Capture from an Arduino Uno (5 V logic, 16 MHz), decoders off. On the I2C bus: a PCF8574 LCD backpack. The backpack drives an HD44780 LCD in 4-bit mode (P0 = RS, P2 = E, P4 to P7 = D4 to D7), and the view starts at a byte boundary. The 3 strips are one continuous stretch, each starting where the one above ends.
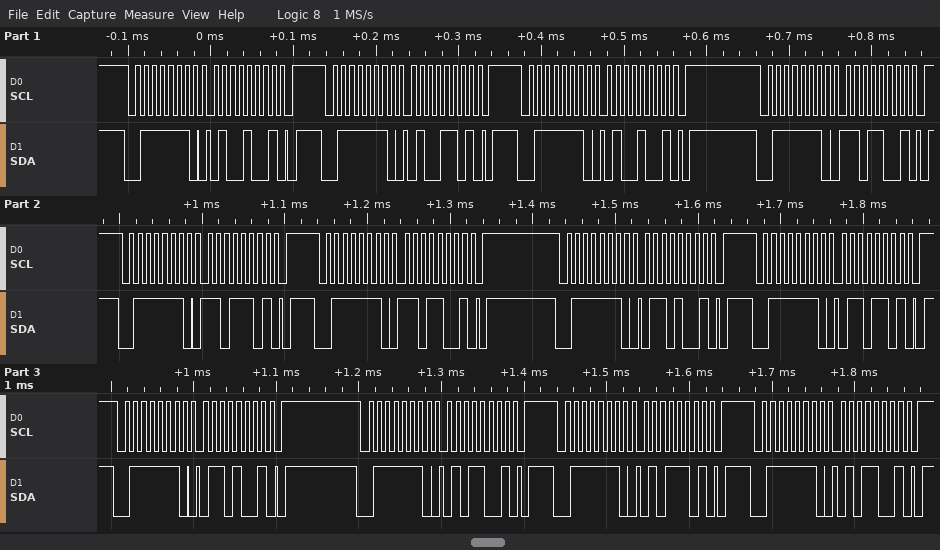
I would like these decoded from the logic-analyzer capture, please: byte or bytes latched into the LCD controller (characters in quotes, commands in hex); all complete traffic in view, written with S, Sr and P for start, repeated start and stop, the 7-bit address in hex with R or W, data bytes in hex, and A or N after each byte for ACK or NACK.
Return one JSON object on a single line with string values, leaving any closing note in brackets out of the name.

{"byte or bytes latched into the LCD controller": "'M' 'e'", "all complete traffic in view, written with S, Sr and P for start, repeated start and stop, the 7-bit address in hex with R or W, data bytes in hex, and A or N after each byte for ACK or NACK": "S 3FW A 49 A P S 3FW A 4D A P S 3FW A 49 A P S 3FW A D9 A P S 3FW A DD A P S 3FW A D9 A P S 3FW A 69 A P S 3FW A 6D A P S 3FW A 69 A P S 3FW A 59 A P S 3FW A 5D A P S 3FW A 59 A P"}
